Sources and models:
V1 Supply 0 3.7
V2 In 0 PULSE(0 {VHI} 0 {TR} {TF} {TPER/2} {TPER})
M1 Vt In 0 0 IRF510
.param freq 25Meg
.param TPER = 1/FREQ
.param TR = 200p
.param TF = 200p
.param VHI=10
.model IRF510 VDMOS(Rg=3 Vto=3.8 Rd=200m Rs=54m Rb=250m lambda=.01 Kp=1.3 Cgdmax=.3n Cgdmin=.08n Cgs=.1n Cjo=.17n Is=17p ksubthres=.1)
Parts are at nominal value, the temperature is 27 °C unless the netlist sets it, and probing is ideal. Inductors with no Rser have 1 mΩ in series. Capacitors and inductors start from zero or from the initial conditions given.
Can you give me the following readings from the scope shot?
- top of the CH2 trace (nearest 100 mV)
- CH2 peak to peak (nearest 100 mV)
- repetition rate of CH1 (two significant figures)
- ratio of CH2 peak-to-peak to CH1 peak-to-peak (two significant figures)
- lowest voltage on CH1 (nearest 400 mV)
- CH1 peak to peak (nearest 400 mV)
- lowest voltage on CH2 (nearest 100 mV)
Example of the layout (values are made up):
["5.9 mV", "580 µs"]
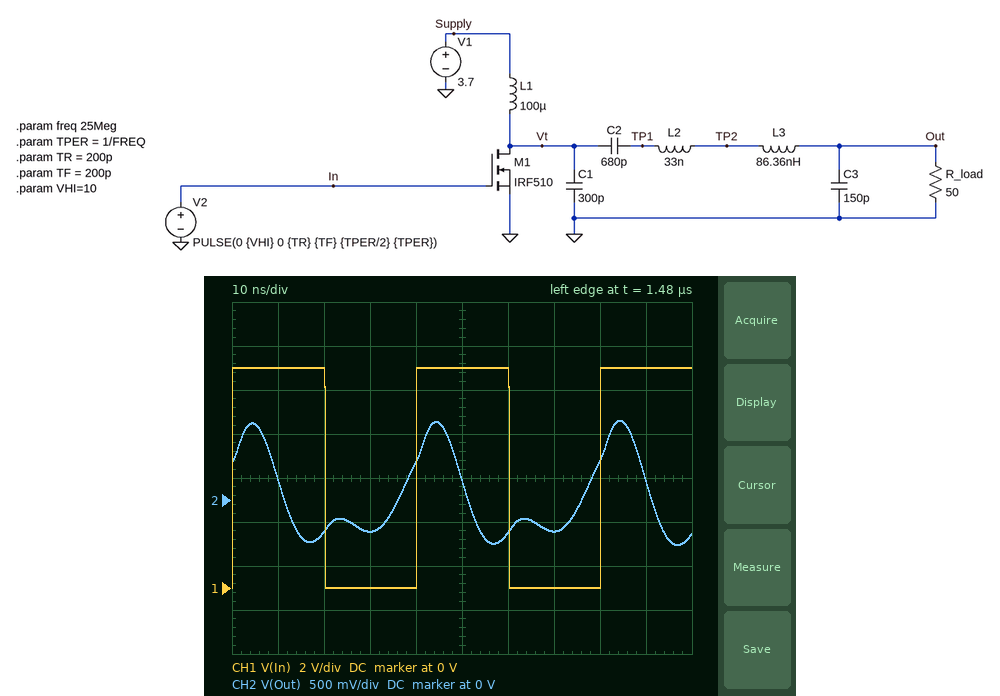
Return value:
["900 mV", "1.4 V", "25 MHz", "0.14", "0 V", "10.0 V", "-500 mV"]
